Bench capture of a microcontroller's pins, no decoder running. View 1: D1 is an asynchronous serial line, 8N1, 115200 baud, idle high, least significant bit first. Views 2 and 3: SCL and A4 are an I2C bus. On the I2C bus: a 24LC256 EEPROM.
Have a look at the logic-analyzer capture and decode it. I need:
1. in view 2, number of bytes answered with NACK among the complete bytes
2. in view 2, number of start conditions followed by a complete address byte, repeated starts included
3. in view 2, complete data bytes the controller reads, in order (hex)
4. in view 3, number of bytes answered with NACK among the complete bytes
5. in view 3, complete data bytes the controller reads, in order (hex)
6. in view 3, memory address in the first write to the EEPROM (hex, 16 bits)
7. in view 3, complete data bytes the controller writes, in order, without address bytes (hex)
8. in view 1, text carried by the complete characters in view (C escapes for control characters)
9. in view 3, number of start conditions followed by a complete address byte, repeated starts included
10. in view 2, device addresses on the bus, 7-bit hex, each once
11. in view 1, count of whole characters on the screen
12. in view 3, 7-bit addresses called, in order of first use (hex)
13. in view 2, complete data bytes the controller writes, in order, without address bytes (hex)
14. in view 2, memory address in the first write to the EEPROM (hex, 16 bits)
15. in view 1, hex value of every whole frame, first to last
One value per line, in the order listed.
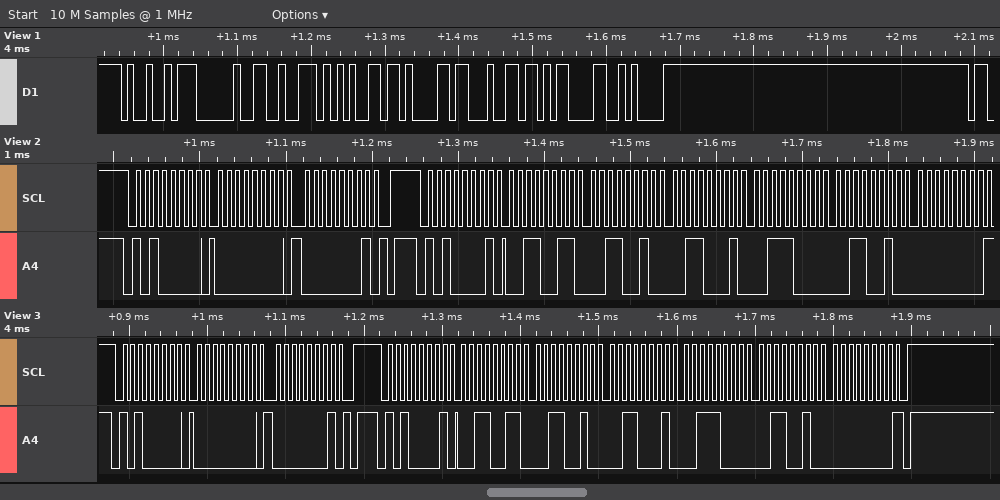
1
2
33 32 31 38 32 00
1
33 32 31 38 32 00
0x0001
00 01
"I read\r\n"
2
0x50
8
0x50
00 01
0x0001
49 20 72 65 61 64 0D 0A
